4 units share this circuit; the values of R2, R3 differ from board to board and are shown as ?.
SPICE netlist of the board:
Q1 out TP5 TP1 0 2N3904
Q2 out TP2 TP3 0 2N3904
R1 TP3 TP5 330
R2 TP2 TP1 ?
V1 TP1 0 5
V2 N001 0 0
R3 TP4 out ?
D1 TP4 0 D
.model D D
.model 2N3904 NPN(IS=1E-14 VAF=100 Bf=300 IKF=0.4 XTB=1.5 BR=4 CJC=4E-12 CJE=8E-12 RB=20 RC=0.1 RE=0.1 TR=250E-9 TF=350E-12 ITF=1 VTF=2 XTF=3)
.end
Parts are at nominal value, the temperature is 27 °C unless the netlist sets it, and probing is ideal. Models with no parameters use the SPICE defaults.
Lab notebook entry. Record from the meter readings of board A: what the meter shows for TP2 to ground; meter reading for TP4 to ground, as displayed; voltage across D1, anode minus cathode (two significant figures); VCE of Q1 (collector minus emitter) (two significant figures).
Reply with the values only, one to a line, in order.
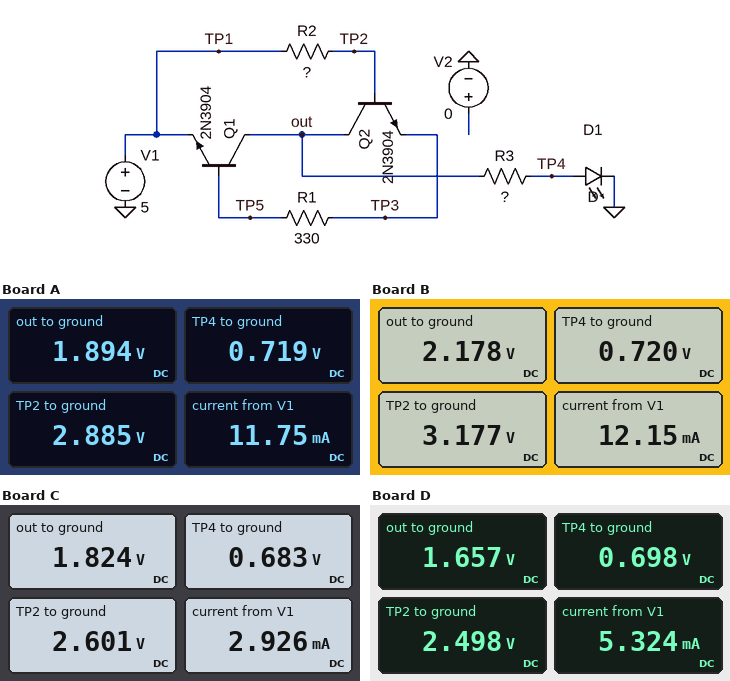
2.885 V
0.719 V
720 mV
-3.1 V
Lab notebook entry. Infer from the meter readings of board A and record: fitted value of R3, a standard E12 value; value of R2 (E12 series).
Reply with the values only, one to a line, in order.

100 Ω
180 Ω
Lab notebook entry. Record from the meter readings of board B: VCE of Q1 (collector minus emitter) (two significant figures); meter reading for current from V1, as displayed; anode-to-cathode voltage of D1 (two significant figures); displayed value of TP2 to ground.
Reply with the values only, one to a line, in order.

-2.8 V
12.15 mA
720 mV
3.177 V
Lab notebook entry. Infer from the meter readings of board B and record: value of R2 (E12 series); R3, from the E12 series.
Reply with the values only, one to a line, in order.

150 Ω
120 Ω
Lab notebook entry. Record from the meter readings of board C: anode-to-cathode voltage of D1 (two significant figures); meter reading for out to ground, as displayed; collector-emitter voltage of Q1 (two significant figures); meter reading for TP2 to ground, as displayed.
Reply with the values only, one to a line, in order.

680 mV
1.824 V
-3.2 V
2.601 V
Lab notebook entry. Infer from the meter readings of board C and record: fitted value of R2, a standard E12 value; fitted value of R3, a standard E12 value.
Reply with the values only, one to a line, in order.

820 Ω
390 Ω
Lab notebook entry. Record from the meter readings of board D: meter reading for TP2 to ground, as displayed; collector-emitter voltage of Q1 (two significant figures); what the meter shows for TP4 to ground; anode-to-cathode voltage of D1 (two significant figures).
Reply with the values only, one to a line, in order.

2.498 V
-3.3 V
0.698 V
700 mV
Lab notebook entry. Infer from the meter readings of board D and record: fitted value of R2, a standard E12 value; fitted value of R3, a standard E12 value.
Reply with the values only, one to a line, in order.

470 Ω
180 Ω
